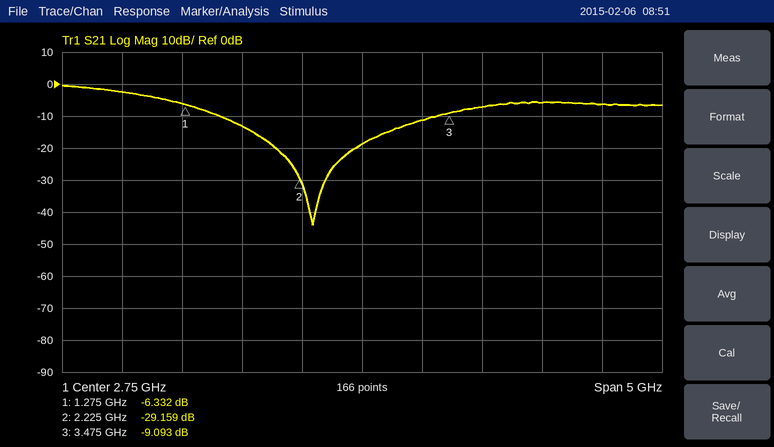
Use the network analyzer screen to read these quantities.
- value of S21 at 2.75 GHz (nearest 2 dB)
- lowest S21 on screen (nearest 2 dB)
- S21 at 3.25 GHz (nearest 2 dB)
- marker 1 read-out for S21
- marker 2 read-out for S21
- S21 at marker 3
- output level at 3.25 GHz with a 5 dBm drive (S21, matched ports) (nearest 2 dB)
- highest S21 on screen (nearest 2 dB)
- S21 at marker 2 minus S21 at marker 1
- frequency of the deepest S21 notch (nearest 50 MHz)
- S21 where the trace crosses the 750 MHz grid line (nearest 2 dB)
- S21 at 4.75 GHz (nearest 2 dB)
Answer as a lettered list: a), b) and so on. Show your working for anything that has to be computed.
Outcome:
a) -18 dB
b) -44 dB
c) -12 dB
d) -6.332 dB
e) -29.159 dB
f) -9.093 dB
g) 5 dBm + (-12 dB) = -6 dBm
h) 0 dB
i) -29.159 − (-6.332) = -22.827 dB
j) 2.35 GHz
k) -2 dB
l) -6 dB
